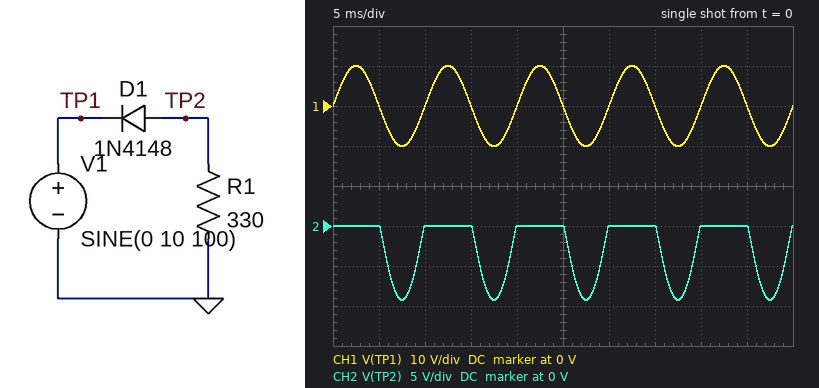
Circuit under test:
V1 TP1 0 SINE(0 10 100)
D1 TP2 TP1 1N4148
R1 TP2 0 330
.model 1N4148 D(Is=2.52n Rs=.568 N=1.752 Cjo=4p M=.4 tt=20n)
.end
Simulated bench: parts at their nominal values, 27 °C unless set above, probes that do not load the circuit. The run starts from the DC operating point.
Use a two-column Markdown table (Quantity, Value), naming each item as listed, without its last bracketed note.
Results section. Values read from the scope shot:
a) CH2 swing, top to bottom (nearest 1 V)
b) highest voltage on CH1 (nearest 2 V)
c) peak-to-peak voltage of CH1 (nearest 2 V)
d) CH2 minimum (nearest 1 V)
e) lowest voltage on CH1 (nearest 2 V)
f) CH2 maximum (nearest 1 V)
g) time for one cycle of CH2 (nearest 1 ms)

| Quantity | Value |
|---|---|
| CH2 swing, top to bottom | 9 V |
| highest voltage on CH1 | 10 V |
| peak-to-peak voltage of CH1 | 20 V |
| CH2 minimum | -9 V |
| lowest voltage on CH1 | -10 V |
| CH2 maximum | 0 V |
| time for one cycle of CH2 | 10 ms |
